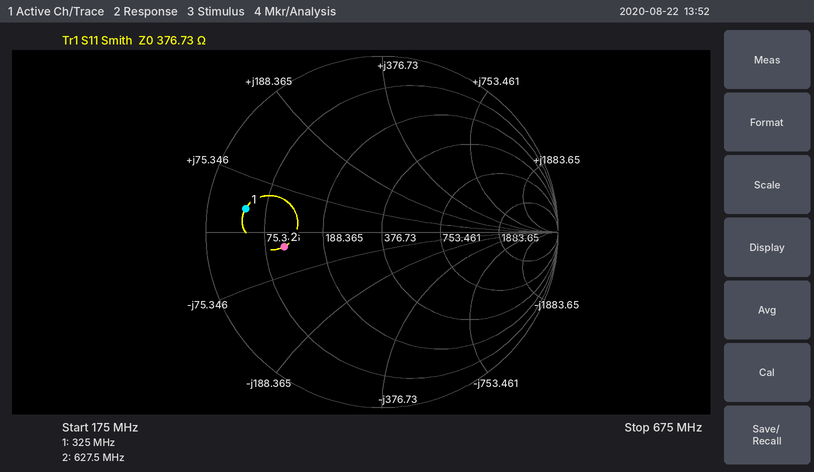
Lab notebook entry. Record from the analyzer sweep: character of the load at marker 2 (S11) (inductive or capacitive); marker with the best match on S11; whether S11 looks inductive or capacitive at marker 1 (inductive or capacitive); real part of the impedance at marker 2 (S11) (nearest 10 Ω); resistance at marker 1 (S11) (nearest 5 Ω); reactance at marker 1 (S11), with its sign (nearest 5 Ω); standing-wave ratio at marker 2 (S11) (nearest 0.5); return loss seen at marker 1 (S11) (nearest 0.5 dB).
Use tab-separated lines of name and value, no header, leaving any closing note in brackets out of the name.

character of the load at marker 2 (S11)	capacitive
marker with the best match on S11	marker 2
whether S11 looks inductive or capacitive at marker 1	inductive
real part of the impedance at marker 2 (S11)	110 Ω
resistance at marker 1 (S11)	45 Ω
reactance at marker 1 (S11), with its sign	+30 Ω
standing-wave ratio at marker 2 (S11)	3.5
return loss seen at marker 1 (S11)	2.0 dB
